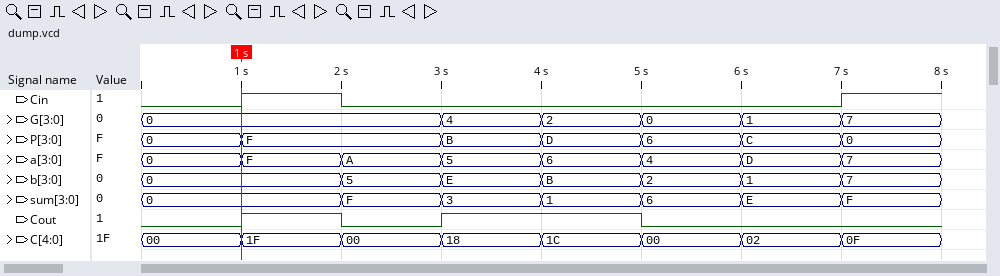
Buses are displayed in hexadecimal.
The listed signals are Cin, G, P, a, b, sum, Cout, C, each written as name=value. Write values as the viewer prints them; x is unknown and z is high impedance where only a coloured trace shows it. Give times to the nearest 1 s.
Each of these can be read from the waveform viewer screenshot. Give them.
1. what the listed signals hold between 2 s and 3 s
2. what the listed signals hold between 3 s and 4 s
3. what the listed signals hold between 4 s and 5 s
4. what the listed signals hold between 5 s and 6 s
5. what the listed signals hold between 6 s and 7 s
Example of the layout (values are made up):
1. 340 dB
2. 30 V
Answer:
1. Cin=0, G=0, P=F, a=A, b=5, sum=F, Cout=0, C=00
2. Cin=0, G=4, P=B, a=5, b=E, sum=3, Cout=1, C=18
3. Cin=0, G=2, P=D, a=6, b=B, sum=1, Cout=1, C=1C
4. Cin=0, G=0, P=6, a=4, b=2, sum=6, Cout=0, C=00
5. Cin=0, G=1, P=C, a=D, b=1, sum=E, Cout=0, C=02
